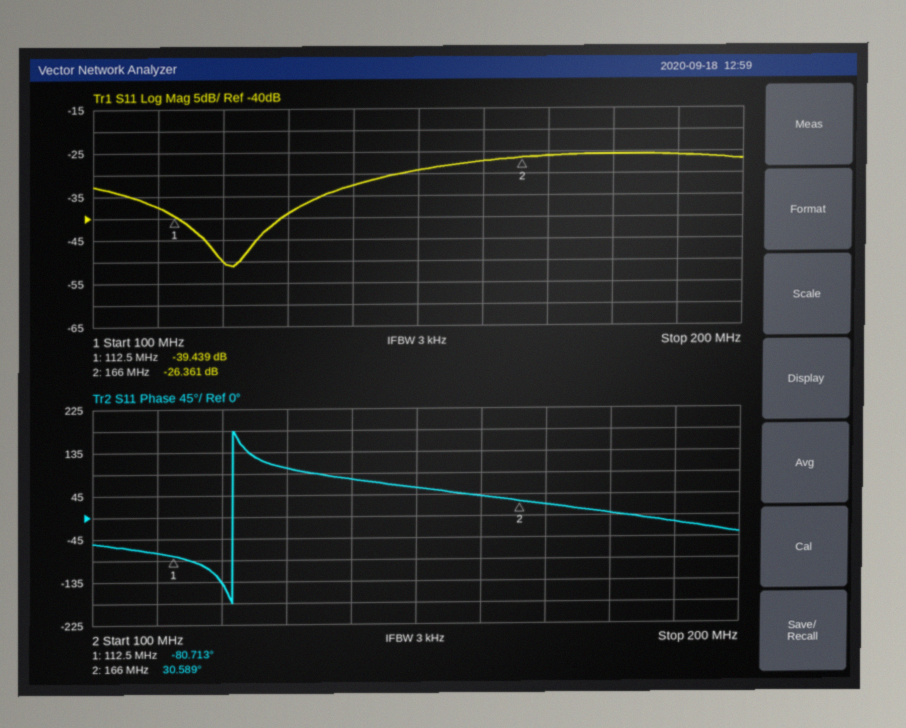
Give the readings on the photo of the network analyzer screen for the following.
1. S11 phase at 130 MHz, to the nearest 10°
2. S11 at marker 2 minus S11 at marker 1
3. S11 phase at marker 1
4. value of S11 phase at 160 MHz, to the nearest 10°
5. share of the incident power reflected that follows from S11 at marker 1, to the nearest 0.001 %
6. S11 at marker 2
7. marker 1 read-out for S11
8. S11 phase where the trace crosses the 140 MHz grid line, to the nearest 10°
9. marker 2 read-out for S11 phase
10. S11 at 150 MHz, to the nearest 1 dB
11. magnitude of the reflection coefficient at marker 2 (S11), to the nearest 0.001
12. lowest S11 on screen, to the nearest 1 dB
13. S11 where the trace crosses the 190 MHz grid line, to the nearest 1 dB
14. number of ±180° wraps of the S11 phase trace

100°
13.078 dB
-80.713°
40°
0.011 %
-26.361 dB
-39.439 dB
80°
30.589°
-29 dB
0.048
-51 dB
-26 dB
1
